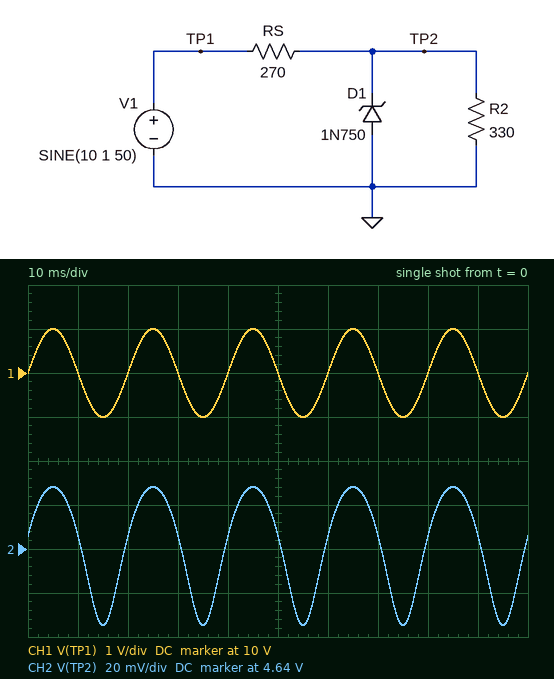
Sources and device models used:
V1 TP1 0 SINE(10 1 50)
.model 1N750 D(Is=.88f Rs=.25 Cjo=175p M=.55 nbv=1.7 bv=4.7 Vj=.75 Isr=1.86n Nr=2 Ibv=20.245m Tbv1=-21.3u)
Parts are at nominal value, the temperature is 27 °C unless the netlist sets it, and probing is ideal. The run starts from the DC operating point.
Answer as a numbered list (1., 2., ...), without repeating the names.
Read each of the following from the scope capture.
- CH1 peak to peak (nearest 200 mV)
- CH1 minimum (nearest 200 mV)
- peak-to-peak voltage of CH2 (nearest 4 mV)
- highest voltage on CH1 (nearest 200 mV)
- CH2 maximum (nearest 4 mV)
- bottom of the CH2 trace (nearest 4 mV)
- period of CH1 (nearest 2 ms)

1. 2.0 V
2. 9.0 V
3. 64 mV
4. 11.0 V
5. 4.668 V
6. 4.604 V
7. 20 ms
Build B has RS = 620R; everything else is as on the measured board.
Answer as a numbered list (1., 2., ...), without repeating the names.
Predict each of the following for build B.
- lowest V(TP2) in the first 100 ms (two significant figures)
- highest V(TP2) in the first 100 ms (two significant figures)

1. 3.1 V
2. 3.8 V
